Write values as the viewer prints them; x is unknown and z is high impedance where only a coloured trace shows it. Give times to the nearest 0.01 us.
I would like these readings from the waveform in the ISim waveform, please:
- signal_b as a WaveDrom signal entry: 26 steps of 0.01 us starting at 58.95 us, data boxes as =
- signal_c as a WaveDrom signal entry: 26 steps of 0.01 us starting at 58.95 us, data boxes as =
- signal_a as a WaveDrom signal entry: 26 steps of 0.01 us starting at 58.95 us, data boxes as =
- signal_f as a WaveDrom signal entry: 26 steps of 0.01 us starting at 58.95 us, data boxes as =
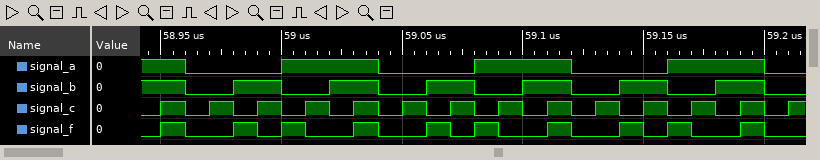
{name: 'signal_b', wave: '10.1.0.1.0.1.0.1.0.1.0.1.0'}
{name: 'signal_c', wave: '10101010101010101010101010'}
{name: 'signal_a', wave: '10...1...0...1...0...1...0'}
{name: 'signal_f', wave: '10.1010.10.1010.10.1010.10'}
